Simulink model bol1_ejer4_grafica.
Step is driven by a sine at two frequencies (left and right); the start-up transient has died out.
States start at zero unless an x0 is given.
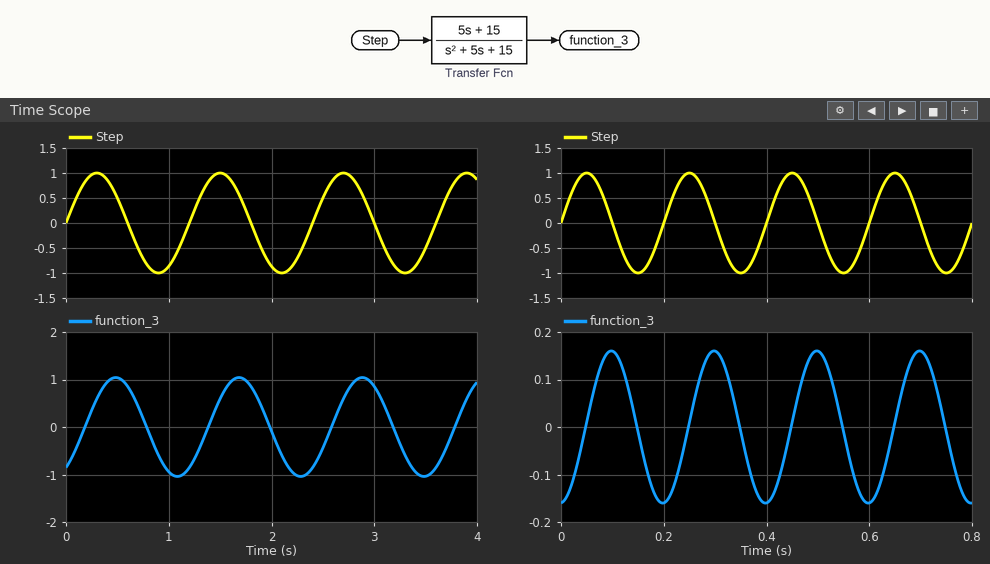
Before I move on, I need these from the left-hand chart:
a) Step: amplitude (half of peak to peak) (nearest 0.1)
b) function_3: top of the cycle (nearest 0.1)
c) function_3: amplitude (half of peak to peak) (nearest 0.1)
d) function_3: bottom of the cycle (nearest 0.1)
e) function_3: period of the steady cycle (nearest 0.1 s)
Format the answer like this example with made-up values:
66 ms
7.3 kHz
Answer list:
1.0
1.0
1.0
-1.0
1.2 s
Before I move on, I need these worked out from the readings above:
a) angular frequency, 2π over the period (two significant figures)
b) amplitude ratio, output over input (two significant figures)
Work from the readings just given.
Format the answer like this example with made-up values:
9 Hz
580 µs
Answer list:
5.2 rad/s
1.0
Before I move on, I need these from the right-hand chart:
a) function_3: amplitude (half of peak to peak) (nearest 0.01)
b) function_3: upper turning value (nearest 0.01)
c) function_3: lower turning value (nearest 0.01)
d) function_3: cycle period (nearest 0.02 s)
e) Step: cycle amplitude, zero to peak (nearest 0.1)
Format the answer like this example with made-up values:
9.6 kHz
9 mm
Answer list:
0.16
0.16
-0.16
0.20 s
1.0
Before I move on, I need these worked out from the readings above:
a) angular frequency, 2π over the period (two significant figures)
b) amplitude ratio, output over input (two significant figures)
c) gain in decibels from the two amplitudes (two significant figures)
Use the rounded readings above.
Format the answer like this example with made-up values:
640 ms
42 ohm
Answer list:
31 rad/s
0.16
-16 dB
